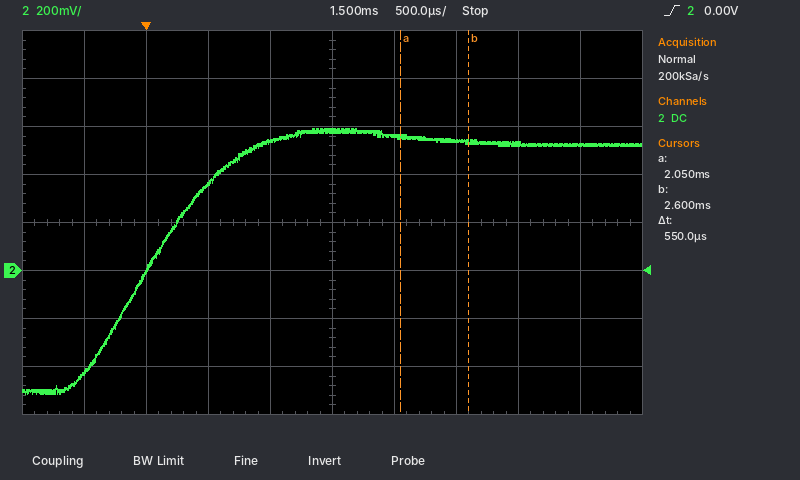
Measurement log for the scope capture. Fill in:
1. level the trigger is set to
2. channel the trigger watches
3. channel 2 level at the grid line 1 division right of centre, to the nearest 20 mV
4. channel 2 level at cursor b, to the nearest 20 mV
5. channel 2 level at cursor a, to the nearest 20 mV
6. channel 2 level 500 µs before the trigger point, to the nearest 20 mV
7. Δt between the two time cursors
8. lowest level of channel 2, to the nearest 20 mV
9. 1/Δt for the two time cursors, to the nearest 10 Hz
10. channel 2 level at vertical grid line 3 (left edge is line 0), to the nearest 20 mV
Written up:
0.00 V
channel 2
560 mV
540 mV
560 mV
-420 mV
550 µs
-520 mV
1.82 kHz
360 mV
